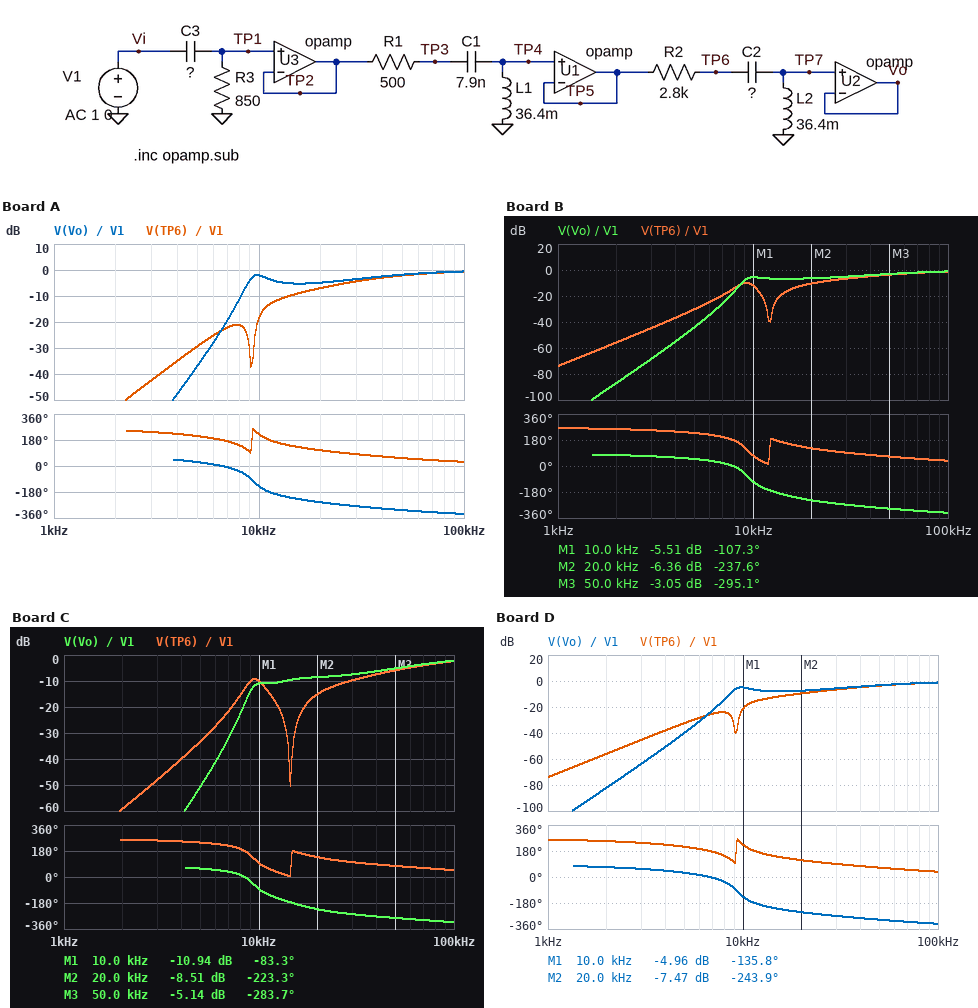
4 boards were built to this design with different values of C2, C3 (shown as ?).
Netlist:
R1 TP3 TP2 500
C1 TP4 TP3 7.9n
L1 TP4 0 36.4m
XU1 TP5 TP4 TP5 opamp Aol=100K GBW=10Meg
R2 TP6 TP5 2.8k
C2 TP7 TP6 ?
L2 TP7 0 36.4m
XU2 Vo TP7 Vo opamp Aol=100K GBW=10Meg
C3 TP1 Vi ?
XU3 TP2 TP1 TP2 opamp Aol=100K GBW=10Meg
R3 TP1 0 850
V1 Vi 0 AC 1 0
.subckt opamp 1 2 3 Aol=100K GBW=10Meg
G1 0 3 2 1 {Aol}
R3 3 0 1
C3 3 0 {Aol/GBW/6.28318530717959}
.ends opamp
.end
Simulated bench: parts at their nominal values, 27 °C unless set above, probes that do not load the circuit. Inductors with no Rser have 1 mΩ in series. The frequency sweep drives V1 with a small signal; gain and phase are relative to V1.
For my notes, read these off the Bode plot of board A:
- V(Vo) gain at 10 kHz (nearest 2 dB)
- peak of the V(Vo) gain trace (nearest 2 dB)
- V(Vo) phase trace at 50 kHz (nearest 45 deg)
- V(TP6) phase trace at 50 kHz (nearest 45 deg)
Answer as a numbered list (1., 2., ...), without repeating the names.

1. -2 dB
2. 0 dB
3. -315 deg
4. 45 deg
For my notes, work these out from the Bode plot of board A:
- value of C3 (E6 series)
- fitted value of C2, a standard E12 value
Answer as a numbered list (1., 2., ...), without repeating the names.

1. 4.7 nF
2. 8.2 nF
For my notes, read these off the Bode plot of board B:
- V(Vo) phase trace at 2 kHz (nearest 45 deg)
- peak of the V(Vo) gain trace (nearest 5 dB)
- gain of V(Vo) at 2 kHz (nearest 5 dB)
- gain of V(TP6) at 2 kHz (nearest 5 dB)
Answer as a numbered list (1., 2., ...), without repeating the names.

1. 90 deg
2. 0 dB
3. -85 dB
4. -55 dB
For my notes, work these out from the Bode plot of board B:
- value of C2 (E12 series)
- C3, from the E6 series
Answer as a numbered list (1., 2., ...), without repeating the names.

1. 4.7 nF
2. 3.3 nF
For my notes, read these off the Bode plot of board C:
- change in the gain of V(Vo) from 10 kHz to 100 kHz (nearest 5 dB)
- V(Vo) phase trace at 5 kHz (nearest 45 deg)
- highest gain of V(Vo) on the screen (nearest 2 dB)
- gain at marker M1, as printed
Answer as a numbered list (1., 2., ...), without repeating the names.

1. 10 dB
2. 45 deg
3. -2 dB
4. -10.94 dB
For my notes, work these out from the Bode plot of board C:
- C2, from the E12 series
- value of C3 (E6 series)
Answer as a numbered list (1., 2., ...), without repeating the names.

1. 3.3 nF
2. 2.2 nF
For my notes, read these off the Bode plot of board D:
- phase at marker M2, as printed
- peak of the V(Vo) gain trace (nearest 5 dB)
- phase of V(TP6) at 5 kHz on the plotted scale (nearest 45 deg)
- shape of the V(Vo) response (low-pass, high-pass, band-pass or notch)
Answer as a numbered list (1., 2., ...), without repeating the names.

1. -243.9 deg
2. 0 dB
3. 225 deg
4. high-pass
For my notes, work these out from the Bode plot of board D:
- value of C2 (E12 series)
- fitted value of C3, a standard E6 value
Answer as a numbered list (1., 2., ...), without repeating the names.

1. 8.2 nF
2. 3.3 nF
